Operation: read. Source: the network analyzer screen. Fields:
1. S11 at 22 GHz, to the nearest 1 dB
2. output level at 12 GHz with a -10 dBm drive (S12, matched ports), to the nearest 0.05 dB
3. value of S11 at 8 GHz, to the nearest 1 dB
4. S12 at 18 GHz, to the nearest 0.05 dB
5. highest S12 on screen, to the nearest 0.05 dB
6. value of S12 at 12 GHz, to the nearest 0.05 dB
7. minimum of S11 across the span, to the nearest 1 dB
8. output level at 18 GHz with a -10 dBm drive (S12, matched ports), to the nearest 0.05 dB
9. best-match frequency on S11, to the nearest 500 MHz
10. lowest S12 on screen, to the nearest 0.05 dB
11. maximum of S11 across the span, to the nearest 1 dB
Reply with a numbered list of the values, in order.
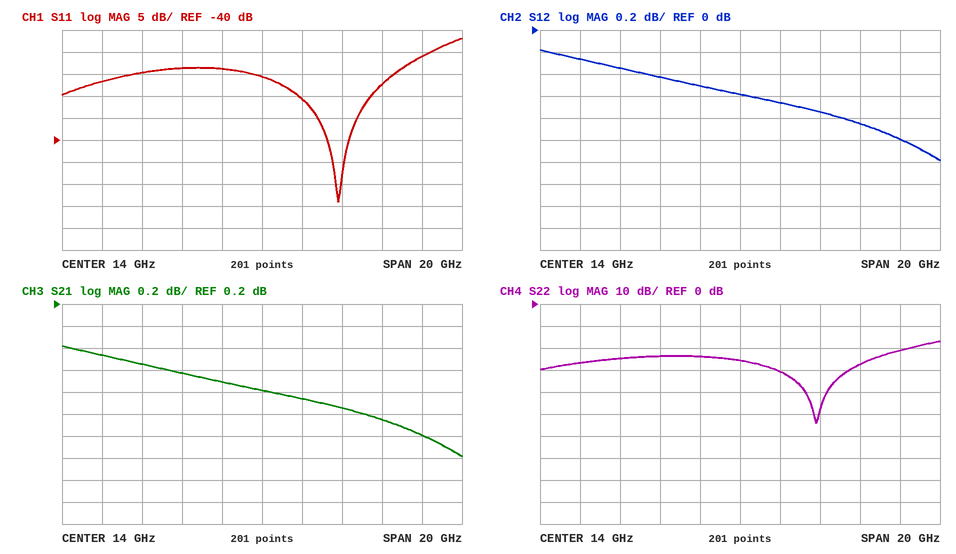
1. -21 dB
2. -10.50 dBm
3. -25 dB
4. -0.75 dB
5. -0.20 dB
6. -0.50 dB
7. -54 dB
8. -10.75 dBm
9. 18.0 GHz
10. -1.20 dB
11. -17 dB
